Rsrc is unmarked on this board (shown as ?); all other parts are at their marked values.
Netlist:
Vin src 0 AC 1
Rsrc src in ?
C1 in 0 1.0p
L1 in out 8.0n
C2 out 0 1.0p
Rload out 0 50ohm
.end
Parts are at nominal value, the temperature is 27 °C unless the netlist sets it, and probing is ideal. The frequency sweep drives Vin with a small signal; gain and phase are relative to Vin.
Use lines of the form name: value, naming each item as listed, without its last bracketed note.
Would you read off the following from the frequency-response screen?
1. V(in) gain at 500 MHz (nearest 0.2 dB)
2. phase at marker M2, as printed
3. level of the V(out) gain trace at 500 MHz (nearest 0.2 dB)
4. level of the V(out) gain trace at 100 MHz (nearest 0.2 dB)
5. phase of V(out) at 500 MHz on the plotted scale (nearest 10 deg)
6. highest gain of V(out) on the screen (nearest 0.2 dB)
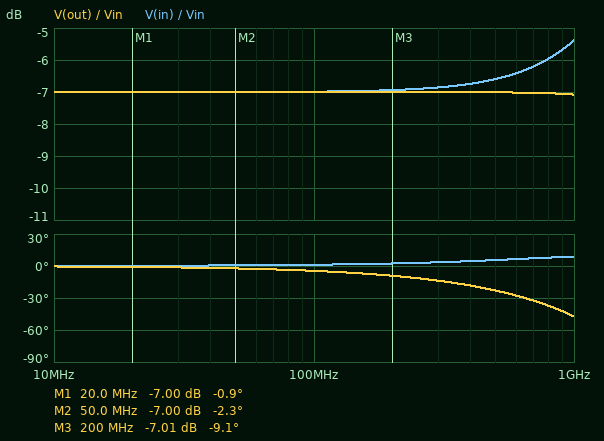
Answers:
V(in) gain at 500 MHz: -6.6 dB
phase at marker M2, as printed: -2.3 deg
level of the V(out) gain trace at 500 MHz: -7.0 dB
level of the V(out) gain trace at 100 MHz: -7.0 dB
phase of V(out) at 500 MHz on the plotted scale: -20 deg
highest gain of V(out) on the screen: -7.0 dB
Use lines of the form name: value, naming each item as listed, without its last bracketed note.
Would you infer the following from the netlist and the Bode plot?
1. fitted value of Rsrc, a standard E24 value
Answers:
fitted value of Rsrc, a standard E24 value: 62 Ω
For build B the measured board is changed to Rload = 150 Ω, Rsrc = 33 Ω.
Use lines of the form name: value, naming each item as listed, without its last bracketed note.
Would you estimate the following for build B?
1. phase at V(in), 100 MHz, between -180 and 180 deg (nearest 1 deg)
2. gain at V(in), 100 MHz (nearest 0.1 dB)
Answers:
phase at V(in), 100 MHz, between -180 and 180 deg: -2 deg
gain at V(in), 100 MHz: -1.7 dB
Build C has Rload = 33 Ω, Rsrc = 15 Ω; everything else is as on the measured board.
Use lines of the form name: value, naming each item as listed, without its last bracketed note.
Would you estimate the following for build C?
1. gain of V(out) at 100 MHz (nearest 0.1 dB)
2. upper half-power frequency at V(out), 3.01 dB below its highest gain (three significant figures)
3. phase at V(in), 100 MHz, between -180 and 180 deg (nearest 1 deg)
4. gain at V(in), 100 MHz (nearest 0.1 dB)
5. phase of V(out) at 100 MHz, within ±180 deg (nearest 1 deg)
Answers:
gain of V(out) at 100 MHz: -3.3 dB
upper half-power frequency at V(out), 3.01 dB below its highest gain: 1.11 GHz
phase at V(in), 100 MHz, between -180 and 180 deg: 2 deg
gain at V(in), 100 MHz: -3.2 dB
phase of V(out) at 100 MHz, within ±180 deg: -7 deg
